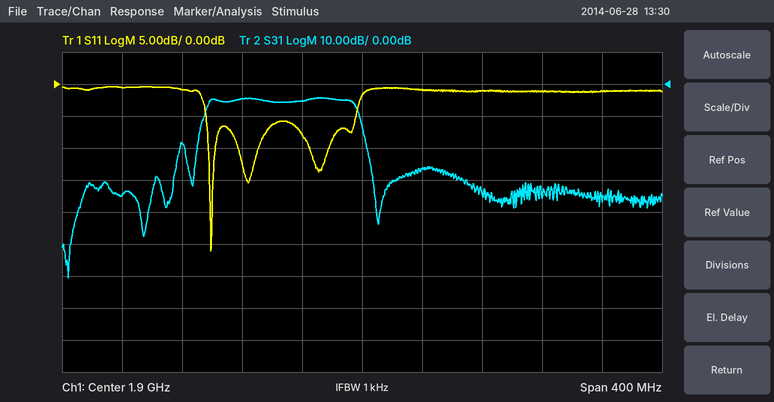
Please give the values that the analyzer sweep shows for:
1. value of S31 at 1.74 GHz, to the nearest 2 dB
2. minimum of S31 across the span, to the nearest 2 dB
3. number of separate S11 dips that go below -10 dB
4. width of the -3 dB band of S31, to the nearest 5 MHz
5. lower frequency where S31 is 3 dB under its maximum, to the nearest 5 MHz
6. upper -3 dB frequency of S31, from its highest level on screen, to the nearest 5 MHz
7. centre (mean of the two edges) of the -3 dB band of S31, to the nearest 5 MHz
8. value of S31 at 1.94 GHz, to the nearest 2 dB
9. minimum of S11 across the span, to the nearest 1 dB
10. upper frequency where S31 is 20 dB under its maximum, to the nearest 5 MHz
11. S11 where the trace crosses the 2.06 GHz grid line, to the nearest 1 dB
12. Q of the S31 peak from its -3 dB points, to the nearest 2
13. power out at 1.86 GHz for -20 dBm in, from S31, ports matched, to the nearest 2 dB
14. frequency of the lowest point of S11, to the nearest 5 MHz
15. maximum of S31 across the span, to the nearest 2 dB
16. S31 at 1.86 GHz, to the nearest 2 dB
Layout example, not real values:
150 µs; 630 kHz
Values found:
-34 dB; -60 dB; 3; 100 MHz; 1.795 GHz; 1.895 GHz; 1.845 GHz; -26 dB; -26 dB; 1.905 GHz; -1 dB; 18; -26 dBm; 1.800 GHz; -4 dB; -6 dB
